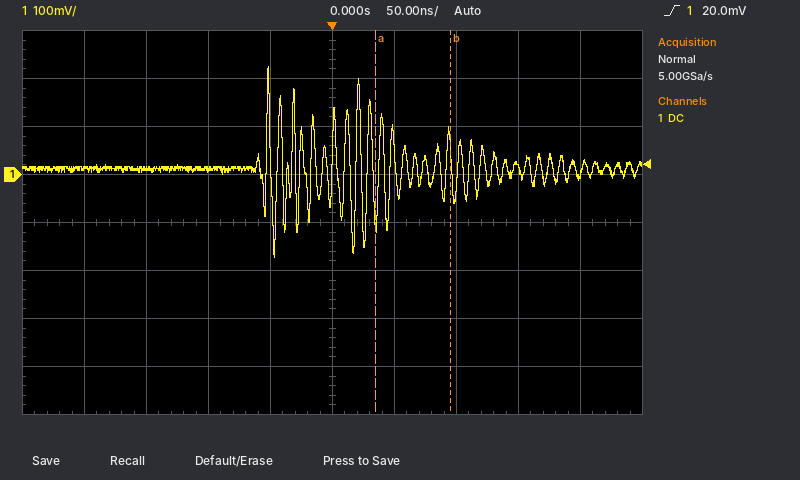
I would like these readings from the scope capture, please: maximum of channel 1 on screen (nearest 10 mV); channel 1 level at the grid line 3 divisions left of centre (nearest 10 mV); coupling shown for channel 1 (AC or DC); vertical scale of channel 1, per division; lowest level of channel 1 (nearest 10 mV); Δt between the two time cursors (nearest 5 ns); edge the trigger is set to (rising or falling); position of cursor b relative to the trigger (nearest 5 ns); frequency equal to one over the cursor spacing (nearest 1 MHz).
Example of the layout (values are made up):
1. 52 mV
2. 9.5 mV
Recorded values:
1. 220 mV
2. 10 mV
3. DC
4. 100 mV
5. -170 mV
6. 60 ns
7. rising
8. +95 ns
9. 17 MHz
